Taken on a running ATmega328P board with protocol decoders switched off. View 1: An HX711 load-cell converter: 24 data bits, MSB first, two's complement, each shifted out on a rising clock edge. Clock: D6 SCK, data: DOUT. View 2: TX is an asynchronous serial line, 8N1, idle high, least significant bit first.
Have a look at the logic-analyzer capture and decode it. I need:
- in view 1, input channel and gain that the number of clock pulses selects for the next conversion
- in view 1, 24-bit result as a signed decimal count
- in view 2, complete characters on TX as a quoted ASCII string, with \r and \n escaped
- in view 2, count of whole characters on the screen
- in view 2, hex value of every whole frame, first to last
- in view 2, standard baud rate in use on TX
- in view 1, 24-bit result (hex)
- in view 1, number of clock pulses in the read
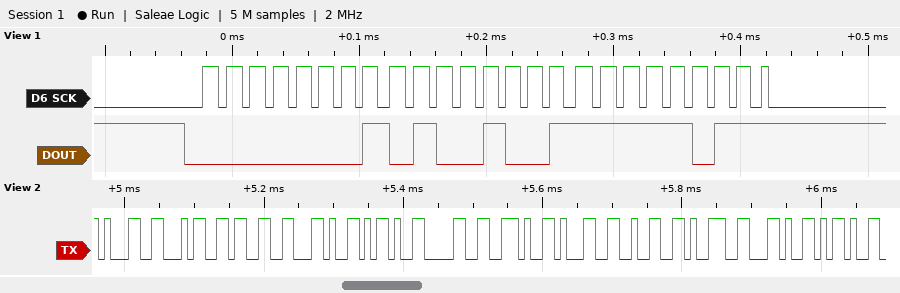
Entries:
channel A, gain 128
84475
"143,-0.129,-"
12
31 34 33 2C 2D 30 2E 31 32 39 2C 2D
115200 baud
0x0149FB
25
